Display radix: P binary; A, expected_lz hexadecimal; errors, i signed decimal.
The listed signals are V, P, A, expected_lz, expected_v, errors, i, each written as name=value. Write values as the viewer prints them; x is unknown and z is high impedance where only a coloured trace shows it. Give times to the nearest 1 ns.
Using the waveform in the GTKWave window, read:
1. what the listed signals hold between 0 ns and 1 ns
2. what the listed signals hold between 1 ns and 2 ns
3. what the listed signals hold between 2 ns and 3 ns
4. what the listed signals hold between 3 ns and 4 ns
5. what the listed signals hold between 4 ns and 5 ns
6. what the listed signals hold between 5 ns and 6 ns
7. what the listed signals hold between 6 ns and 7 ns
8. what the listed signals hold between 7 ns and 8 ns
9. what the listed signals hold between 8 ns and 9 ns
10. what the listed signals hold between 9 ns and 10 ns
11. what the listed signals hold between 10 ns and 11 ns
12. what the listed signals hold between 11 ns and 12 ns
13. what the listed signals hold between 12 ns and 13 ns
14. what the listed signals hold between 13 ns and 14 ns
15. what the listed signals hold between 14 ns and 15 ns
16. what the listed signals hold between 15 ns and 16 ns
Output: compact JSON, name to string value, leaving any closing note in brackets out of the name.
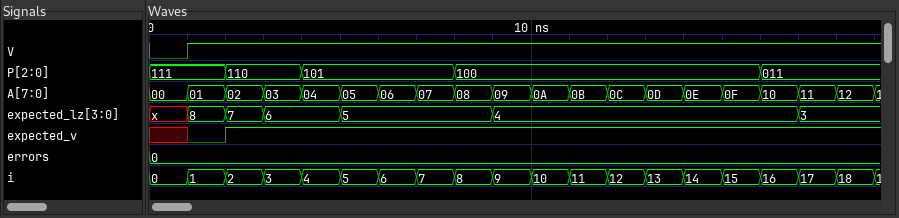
{"what the listed signals hold between 0 ns and 1 ns": "V=0, P=111, A=00, expected_lz=x, expected_v=x, errors=0, i=0", "what the listed signals hold between 1 ns and 2 ns": "V=1, P=111, A=01, expected_lz=8, expected_v=0, errors=0, i=1", "what the listed signals hold between 2 ns and 3 ns": "V=1, P=110, A=02, expected_lz=7, expected_v=1, errors=0, i=2", "what the listed signals hold between 3 ns and 4 ns": "V=1, P=110, A=03, expected_lz=6, expected_v=1, errors=0, i=3", "what the listed signals hold between 4 ns and 5 ns": "V=1, P=101, A=04, expected_lz=6, expected_v=1, errors=0, i=4", "what the listed signals hold between 5 ns and 6 ns": "V=1, P=101, A=05, expected_lz=5, expected_v=1, errors=0, i=5", "what the listed signals hold between 6 ns and 7 ns": "V=1, P=101, A=06, expected_lz=5, expected_v=1, errors=0, i=6", "what the listed signals hold between 7 ns and 8 ns": "V=1, P=101, A=07, expected_lz=5, expected_v=1, errors=0, i=7", "what the listed signals hold between 8 ns and 9 ns": "V=1, P=100, A=08, expected_lz=5, expected_v=1, errors=0, i=8", "what the listed signals hold between 9 ns and 10 ns": "V=1, P=100, A=09, expected_lz=4, expected_v=1, errors=0, i=9", "what the listed signals hold between 10 ns and 11 ns": "V=1, P=100, A=0A, expected_lz=4, expected_v=1, errors=0, i=10", "what the listed signals hold between 11 ns and 12 ns": "V=1, P=100, A=0B, expected_lz=4, expected_v=1, errors=0, i=11", "what the listed signals hold between 12 ns and 13 ns": "V=1, P=100, A=0C, expected_lz=4, expected_v=1, errors=0, i=12", "what the listed signals hold between 13 ns and 14 ns": "V=1, P=100, A=0D, expected_lz=4, expected_v=1, errors=0, i=13", "what the listed signals hold between 14 ns and 15 ns": "V=1, P=100, A=0E, expected_lz=4, expected_v=1, errors=0, i=14", "what the listed signals hold between 15 ns and 16 ns": "V=1, P=100, A=0F, expected_lz=4, expected_v=1, errors=0, i=15"}
